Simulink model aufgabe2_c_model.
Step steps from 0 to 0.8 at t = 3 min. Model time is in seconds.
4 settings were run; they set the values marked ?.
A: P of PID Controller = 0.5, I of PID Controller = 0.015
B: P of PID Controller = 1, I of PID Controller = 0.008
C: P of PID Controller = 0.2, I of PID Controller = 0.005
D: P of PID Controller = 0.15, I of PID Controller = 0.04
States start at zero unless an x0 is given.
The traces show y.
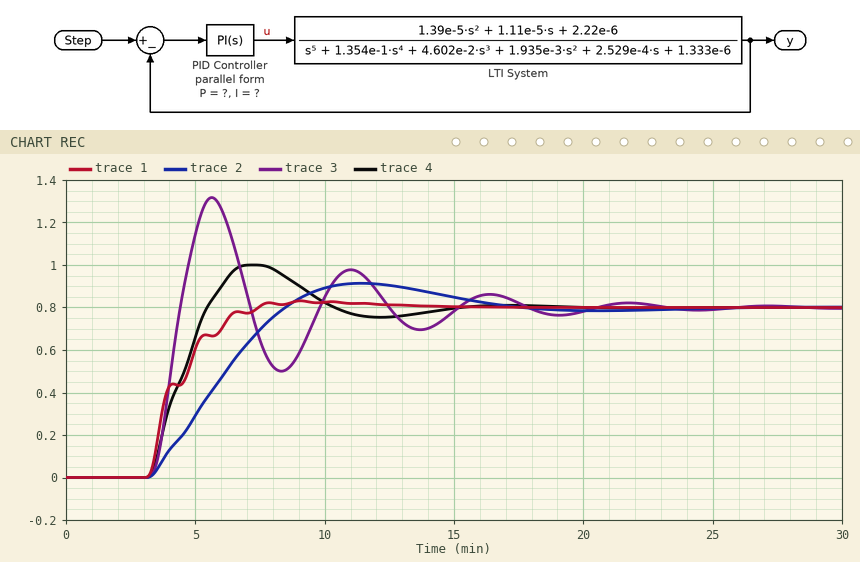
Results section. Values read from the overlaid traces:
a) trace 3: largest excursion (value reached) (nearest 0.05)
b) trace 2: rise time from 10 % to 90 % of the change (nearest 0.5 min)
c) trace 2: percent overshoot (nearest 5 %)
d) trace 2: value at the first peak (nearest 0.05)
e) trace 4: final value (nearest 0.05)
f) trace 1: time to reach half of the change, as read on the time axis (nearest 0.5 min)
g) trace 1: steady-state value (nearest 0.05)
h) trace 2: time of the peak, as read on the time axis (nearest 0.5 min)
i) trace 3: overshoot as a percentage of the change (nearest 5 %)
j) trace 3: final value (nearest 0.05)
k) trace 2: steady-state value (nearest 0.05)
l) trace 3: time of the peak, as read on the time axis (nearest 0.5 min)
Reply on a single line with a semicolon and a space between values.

1.30; 4.0 min; 15 %; 0.90; 0.80; 4.0 min; 0.80; 11.5 min; 65 %; 0.80; 0.80; 5.5 min
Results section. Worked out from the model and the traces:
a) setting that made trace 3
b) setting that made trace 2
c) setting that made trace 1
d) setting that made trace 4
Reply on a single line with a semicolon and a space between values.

D; C; B; A
